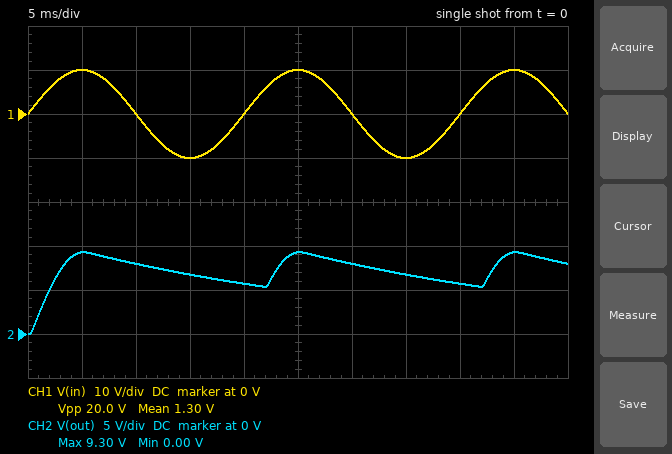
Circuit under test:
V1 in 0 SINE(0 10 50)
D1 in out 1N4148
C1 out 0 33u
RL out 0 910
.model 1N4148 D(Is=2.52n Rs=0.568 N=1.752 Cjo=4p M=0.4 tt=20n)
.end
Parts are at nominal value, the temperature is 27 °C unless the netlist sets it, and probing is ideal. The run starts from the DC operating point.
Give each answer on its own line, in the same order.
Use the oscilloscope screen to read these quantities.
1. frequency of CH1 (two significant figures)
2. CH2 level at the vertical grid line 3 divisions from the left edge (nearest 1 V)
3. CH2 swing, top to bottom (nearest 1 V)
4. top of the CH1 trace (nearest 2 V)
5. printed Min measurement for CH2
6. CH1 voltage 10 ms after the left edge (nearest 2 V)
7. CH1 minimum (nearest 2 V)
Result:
50 Hz
7 V
9 V
10 V
0.00 V
0 V
-10 V
